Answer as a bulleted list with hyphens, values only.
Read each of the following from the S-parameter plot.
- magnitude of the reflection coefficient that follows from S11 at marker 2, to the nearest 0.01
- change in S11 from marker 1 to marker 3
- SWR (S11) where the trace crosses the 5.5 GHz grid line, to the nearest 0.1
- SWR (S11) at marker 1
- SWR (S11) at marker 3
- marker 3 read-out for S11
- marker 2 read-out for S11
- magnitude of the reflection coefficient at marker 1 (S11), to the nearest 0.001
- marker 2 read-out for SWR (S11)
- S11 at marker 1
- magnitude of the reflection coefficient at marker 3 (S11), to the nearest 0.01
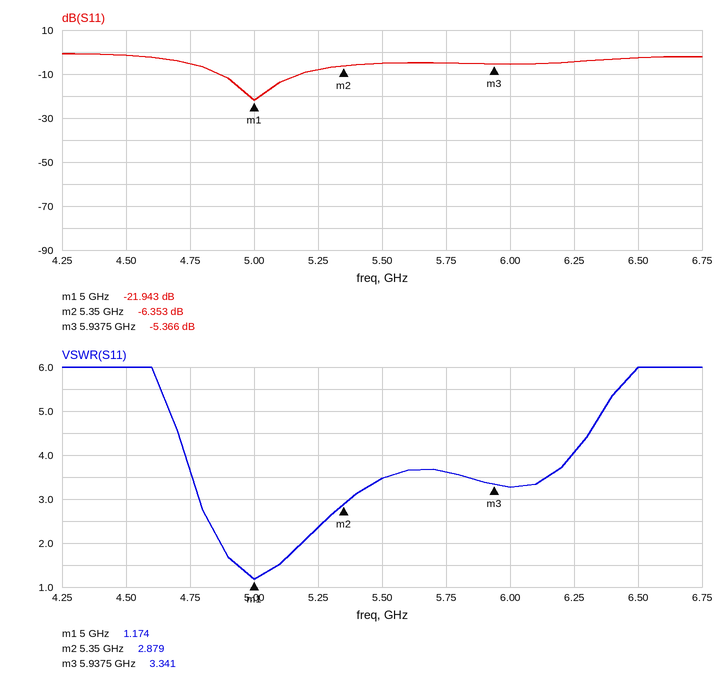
- 0.48
- 16.577 dB
- 3.5
- 1.174
- 3.341
- -5.366 dB
- -6.353 dB
- 0.080
- 2.879
- -21.943 dB
- 0.54
